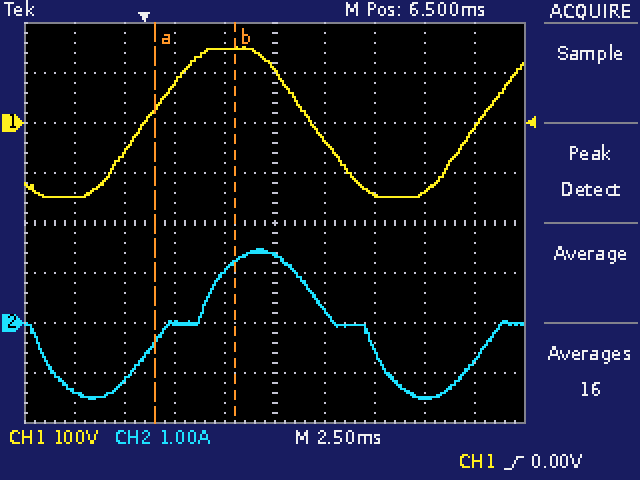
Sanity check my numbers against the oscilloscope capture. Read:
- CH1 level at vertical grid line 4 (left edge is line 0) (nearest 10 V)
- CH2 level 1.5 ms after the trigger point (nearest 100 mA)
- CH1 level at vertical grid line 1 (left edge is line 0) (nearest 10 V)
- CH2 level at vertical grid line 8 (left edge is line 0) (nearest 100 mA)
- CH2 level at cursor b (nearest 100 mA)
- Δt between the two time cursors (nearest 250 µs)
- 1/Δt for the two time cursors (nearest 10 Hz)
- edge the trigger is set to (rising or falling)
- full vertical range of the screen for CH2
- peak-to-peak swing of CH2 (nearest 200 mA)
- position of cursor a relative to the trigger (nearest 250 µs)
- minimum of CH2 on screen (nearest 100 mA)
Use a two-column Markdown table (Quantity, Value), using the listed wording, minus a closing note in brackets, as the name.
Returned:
| Quantity | Value |
|---|---|
| CH1 level at vertical grid line 4 (left edge is line 0) | 150 V |
| CH2 level 1.5 ms after the trigger point | 0.0 A |
| CH1 level at vertical grid line 1 (left edge is line 0) | -150 V |
| CH2 level at vertical grid line 8 (left edge is line 0) | -1.5 A |
| CH2 level at cursor b | 1.2 A |
| Δt between the two time cursors | 4.00 ms |
| 1/Δt for the two time cursors | 250 Hz |
| edge the trigger is set to | rising |
| full vertical range of the screen for CH2 | 8 A |
| peak-to-peak swing of CH2 | 3.0 A |
| position of cursor a relative to the trigger | +500 µs |
| minimum of CH2 on screen | -1.5 A |
